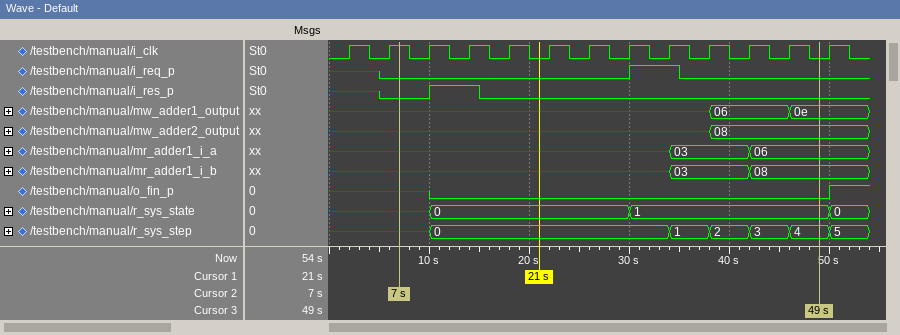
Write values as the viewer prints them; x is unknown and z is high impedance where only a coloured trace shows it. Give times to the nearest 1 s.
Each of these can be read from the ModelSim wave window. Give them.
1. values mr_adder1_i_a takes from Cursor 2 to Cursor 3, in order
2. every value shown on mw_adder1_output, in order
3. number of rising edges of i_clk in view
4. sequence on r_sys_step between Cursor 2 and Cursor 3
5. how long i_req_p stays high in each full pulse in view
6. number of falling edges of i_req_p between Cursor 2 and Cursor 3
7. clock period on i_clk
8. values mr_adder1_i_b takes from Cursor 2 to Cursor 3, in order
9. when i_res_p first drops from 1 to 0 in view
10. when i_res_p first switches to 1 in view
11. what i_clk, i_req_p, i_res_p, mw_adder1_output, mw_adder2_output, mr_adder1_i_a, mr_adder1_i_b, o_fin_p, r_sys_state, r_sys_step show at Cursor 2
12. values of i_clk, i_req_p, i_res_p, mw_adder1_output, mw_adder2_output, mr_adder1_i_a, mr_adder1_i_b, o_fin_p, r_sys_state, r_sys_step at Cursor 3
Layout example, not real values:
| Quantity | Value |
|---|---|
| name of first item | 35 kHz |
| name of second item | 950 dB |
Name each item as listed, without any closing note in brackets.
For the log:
| Quantity | Value |
|---|---|
| values mr_adder1_i_a takes from Cursor 2 to Cursor 3, in order | x, 03, 06 |
| every value shown on mw_adder1_output, in order | x, 06, 0e |
| number of rising edges of i_clk in view | 13 |
| sequence on r_sys_step between Cursor 2 and Cursor 3 | x, 0, 1, 2, 3, 4 |
| how long i_req_p stays high in each full pulse in view | 5 s |
| number of falling edges of i_req_p between Cursor 2 and Cursor 3 | 1 |
| clock period on i_clk | 4 s |
| values mr_adder1_i_b takes from Cursor 2 to Cursor 3, in order | x, 03, 08 |
| when i_res_p first drops from 1 to 0 in view | 15 s |
| when i_res_p first switches to 1 in view | 10 s |
| what i_clk, i_req_p, i_res_p, mw_adder1_output, mw_adder2_output, mr_adder1_i_a, mr_adder1_i_b, o_fin_p, r_sys_state, r_sys_step show at Cursor 2 | i_clk=1, i_req_p=0, i_res_p=0, mw_adder1_output=x, mw_adder2_output=x, mr_adder1_i_a=x, mr_adder1_i_b=x, o_fin_p=x, r_sys_state=x, r_sys_step=x |
| values of i_clk, i_req_p, i_res_p, mw_adder1_output, mw_adder2_output, mr_adder1_i_a, mr_adder1_i_b, o_fin_p, r_sys_state, r_sys_step at Cursor 3 | i_clk=0, i_req_p=0, i_res_p=0, mw_adder1_output=0e, mw_adder2_output=08, mr_adder1_i_a=06, mr_adder1_i_b=08, o_fin_p=0, r_sys_state=1, r_sys_step=4 |
